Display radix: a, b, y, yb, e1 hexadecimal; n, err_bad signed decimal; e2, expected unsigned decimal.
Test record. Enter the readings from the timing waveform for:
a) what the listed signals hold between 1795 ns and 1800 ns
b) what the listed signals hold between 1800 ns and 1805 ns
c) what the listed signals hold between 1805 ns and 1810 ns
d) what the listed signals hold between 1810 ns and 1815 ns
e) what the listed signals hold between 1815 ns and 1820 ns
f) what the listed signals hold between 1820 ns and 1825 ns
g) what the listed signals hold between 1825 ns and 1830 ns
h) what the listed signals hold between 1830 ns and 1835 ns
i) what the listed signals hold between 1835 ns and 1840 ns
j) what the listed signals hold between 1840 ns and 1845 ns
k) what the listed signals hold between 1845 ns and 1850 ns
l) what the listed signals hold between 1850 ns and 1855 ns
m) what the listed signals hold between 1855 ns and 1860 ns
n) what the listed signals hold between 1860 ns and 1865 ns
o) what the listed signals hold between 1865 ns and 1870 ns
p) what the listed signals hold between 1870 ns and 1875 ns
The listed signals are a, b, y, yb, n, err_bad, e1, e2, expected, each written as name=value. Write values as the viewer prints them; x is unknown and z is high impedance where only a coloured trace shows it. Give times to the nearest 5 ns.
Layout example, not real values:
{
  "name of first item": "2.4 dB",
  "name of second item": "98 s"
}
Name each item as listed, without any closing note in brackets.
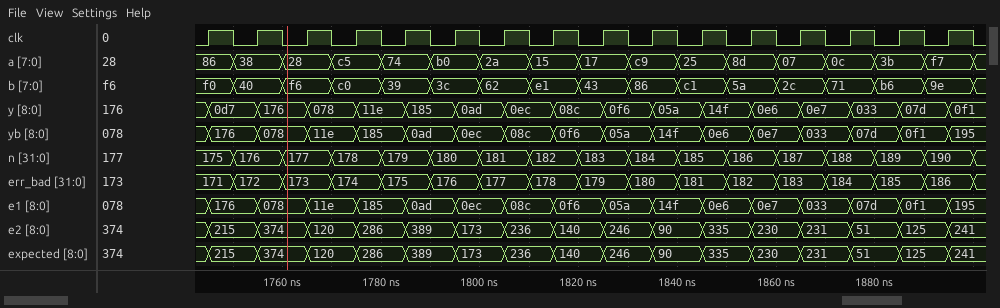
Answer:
{
  "what the listed signals hold between 1795 ns and 1800 ns": "a=b0, b=3c, y=0ad, yb=0ec, n=180, err_bad=176, e1=0ec, e2=173, expected=173",
  "what the listed signals hold between 1800 ns and 1805 ns": "a=2a, b=62, y=0ad, yb=0ec, n=181, err_bad=177, e1=0ec, e2=173, expected=173",
  "what the listed signals hold between 1805 ns and 1810 ns": "a=2a, b=62, y=0ec, yb=08c, n=181, err_bad=177, e1=08c, e2=236, expected=236",
  "what the listed signals hold between 1810 ns and 1815 ns": "a=15, b=e1, y=0ec, yb=08c, n=182, err_bad=178, e1=08c, e2=236, expected=236",
  "what the listed signals hold between 1815 ns and 1820 ns": "a=15, b=e1, y=08c, yb=0f6, n=182, err_bad=178, e1=0f6, e2=140, expected=140",
  "what the listed signals hold between 1820 ns and 1825 ns": "a=17, b=43, y=08c, yb=0f6, n=183, err_bad=179, e1=0f6, e2=140, expected=140",
  "what the listed signals hold between 1825 ns and 1830 ns": "a=17, b=43, y=0f6, yb=05a, n=183, err_bad=179, e1=05a, e2=246, expected=246",
  "what the listed signals hold between 1830 ns and 1835 ns": "a=c9, b=86, y=0f6, yb=05a, n=184, err_bad=180, e1=05a, e2=246, expected=246",
  "what the listed signals hold between 1835 ns and 1840 ns": "a=c9, b=86, y=05a, yb=14f, n=184, err_bad=180, e1=14f, e2=90, expected=90",
  "what the listed signals hold between 1840 ns and 1845 ns": "a=25, b=c1, y=05a, yb=14f, n=185, err_bad=181, e1=14f, e2=90, expected=90",
  "what the listed signals hold between 1845 ns and 1850 ns": "a=25, b=c1, y=14f, yb=0e6, n=185, err_bad=181, e1=0e6, e2=335, expected=335",
  "what the listed signals hold between 1850 ns and 1855 ns": "a=8d, b=5a, y=14f, yb=0e6, n=186, err_bad=182, e1=0e6, e2=335, expected=335",
  "what the listed signals hold between 1855 ns and 1860 ns": "a=8d, b=5a, y=0e6, yb=0e7, n=186, err_bad=182, e1=0e7, e2=230, expected=230",
  "what the listed signals hold between 1860 ns and 1865 ns": "a=07, b=2c, y=0e6, yb=0e7, n=187, err_bad=183, e1=0e7, e2=230, expected=230",
  "what the listed signals hold between 1865 ns and 1870 ns": "a=07, b=2c, y=0e7, yb=033, n=187, err_bad=183, e1=033, e2=231, expected=231",
  "what the listed signals hold between 1870 ns and 1875 ns": "a=0c, b=71, y=0e7, yb=033, n=188, err_bad=184, e1=033, e2=231, expected=231"
}
